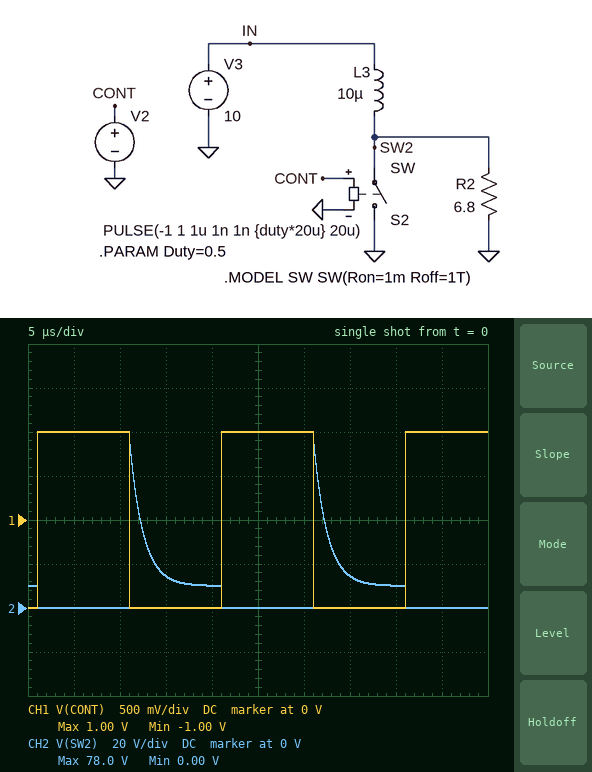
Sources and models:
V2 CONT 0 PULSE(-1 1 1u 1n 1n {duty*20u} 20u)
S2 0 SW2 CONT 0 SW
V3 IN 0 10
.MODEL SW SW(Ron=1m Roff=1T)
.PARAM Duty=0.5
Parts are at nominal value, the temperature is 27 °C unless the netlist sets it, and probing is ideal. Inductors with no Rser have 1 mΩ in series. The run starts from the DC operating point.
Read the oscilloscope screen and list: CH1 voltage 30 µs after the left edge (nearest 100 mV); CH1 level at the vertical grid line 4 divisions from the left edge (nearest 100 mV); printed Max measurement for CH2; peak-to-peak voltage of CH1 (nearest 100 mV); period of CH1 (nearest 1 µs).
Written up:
1.0 V
-1.0 V
78.0 V
2.0 V
20 µs
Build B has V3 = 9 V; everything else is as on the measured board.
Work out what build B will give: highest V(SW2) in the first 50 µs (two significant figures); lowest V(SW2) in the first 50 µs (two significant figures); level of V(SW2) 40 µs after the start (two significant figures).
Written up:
70 V
1.3 mV
9.1 V
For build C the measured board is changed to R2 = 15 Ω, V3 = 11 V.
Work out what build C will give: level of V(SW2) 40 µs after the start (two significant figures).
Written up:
11 V
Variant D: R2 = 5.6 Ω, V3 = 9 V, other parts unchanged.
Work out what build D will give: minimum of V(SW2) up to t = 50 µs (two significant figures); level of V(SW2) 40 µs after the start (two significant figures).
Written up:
1.6 mV
9.3 V
